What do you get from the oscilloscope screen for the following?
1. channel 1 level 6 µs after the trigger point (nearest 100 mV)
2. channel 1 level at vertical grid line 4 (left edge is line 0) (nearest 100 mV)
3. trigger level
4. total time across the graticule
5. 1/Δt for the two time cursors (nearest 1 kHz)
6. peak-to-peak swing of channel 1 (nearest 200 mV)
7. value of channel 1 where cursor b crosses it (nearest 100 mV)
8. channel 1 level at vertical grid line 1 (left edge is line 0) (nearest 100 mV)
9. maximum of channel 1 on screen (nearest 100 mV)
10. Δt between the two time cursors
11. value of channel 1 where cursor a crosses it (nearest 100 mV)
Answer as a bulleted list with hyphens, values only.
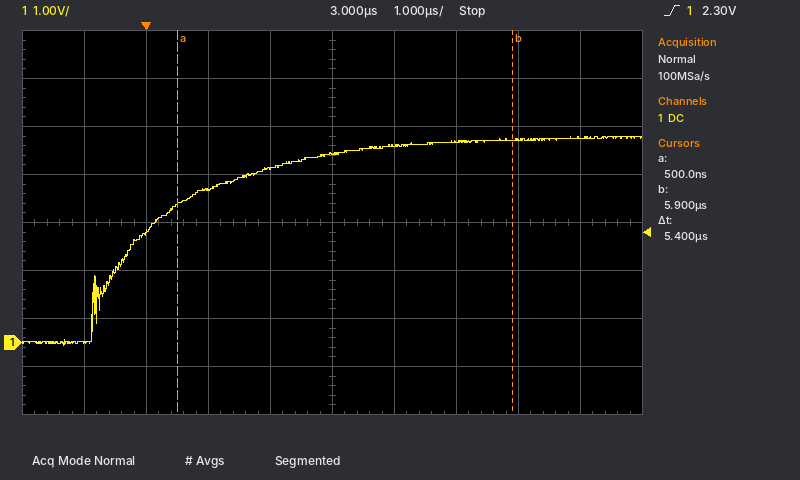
- 4.2 V
- 3.6 V
- 2.30 V
- 10 µs
- 185 kHz
- 4.4 V
- 4.2 V
- 0.0 V
- 4.3 V
- 5.4 µs
- 2.9 V
